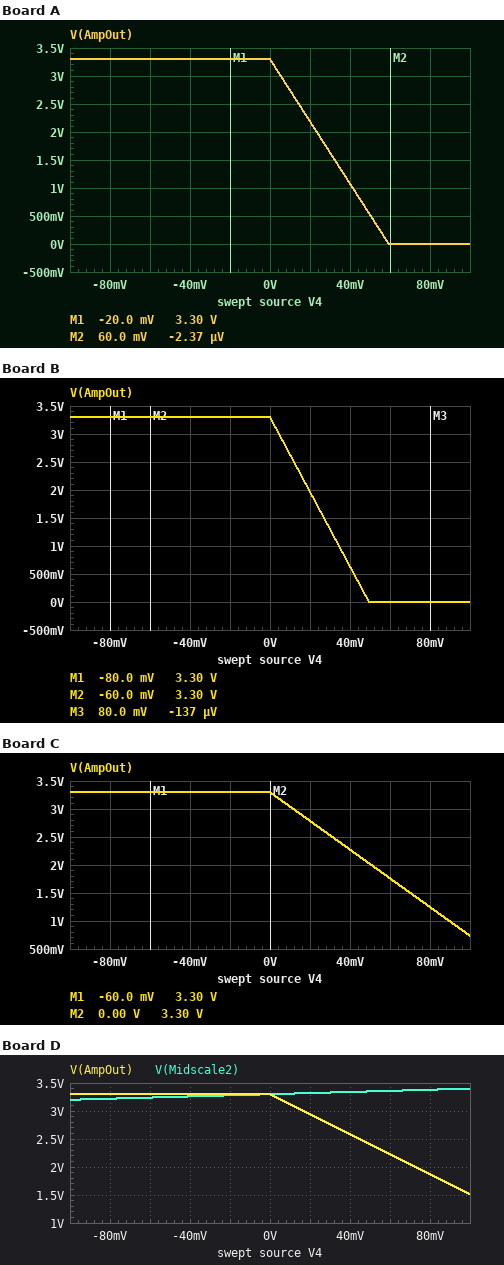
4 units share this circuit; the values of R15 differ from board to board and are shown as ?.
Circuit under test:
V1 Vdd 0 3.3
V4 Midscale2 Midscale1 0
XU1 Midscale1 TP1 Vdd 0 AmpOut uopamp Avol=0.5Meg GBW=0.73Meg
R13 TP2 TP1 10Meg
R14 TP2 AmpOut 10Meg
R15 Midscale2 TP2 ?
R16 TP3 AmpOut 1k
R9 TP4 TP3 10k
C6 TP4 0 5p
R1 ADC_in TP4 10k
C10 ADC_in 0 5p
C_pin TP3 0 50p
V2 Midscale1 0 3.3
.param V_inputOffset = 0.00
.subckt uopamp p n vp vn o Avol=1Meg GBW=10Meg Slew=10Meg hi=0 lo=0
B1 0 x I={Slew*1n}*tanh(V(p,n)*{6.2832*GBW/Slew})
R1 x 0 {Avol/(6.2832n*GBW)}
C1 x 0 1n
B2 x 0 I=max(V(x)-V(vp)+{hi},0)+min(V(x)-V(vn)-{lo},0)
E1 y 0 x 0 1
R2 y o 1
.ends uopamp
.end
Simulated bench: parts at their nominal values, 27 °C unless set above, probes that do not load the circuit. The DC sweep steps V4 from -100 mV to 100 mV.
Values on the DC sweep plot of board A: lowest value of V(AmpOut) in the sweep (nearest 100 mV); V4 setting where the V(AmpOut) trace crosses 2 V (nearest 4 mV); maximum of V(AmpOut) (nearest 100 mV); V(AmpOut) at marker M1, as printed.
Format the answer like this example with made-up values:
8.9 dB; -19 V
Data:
0 V; 24 mV; 3.3 V; 3.30 V
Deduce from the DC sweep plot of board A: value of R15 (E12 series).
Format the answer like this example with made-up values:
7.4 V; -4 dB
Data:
180 kΩ
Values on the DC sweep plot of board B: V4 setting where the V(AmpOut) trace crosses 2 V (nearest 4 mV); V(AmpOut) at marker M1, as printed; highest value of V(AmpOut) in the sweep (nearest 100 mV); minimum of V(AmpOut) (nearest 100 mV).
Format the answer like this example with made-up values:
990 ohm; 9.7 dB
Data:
20 mV; 3.30 V; 3.3 V; 0 V
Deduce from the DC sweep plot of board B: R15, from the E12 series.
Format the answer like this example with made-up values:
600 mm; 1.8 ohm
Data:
150 kΩ
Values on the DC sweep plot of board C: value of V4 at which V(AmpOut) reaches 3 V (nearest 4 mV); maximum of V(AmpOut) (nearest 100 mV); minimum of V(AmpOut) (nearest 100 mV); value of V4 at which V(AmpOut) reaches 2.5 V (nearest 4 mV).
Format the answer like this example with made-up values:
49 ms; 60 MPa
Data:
12 mV; 3.3 V; 700 mV; 32 mV
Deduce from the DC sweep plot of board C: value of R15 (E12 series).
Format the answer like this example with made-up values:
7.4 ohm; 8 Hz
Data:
390 kΩ
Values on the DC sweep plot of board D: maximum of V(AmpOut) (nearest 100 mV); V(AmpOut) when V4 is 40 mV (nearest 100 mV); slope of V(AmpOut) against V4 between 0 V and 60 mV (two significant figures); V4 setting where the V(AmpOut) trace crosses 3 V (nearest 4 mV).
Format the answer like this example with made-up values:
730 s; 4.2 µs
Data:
3.3 V; 2.6 V; -18 V/V; 16 mV
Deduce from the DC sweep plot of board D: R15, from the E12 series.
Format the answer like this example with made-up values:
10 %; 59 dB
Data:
560 kΩ
